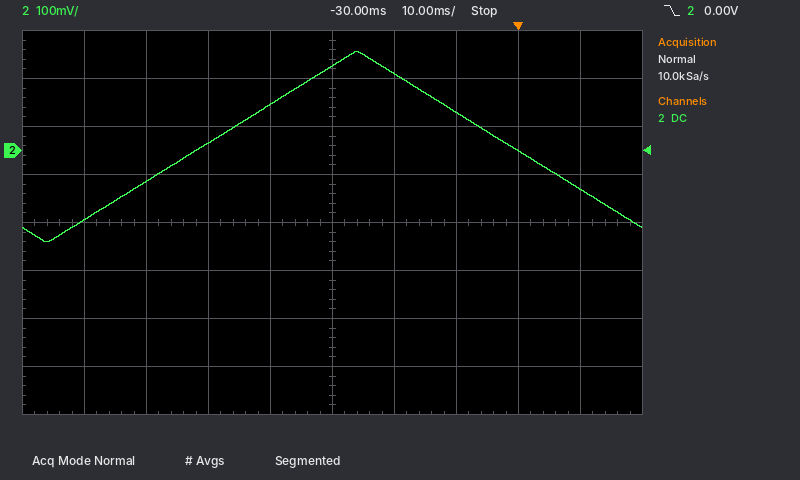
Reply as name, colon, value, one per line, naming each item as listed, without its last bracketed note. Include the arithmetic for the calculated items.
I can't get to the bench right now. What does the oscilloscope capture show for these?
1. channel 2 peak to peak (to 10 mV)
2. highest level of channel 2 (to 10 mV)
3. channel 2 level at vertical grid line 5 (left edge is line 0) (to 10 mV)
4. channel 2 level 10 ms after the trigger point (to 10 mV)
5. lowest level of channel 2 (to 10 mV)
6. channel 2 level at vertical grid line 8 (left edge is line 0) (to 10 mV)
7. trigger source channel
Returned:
channel 2 peak to peak: 210 mV − (-190 mV) = 400 mV
highest level of channel 2: 210 mV
channel 2 level at vertical grid line 5 (left edge is line 0): 180 mV
channel 2 level 10 ms after the trigger point: -80 mV
lowest level of channel 2: -190 mV
channel 2 level at vertical grid line 8 (left edge is line 0): 0 mV
trigger source channel: channel 2
